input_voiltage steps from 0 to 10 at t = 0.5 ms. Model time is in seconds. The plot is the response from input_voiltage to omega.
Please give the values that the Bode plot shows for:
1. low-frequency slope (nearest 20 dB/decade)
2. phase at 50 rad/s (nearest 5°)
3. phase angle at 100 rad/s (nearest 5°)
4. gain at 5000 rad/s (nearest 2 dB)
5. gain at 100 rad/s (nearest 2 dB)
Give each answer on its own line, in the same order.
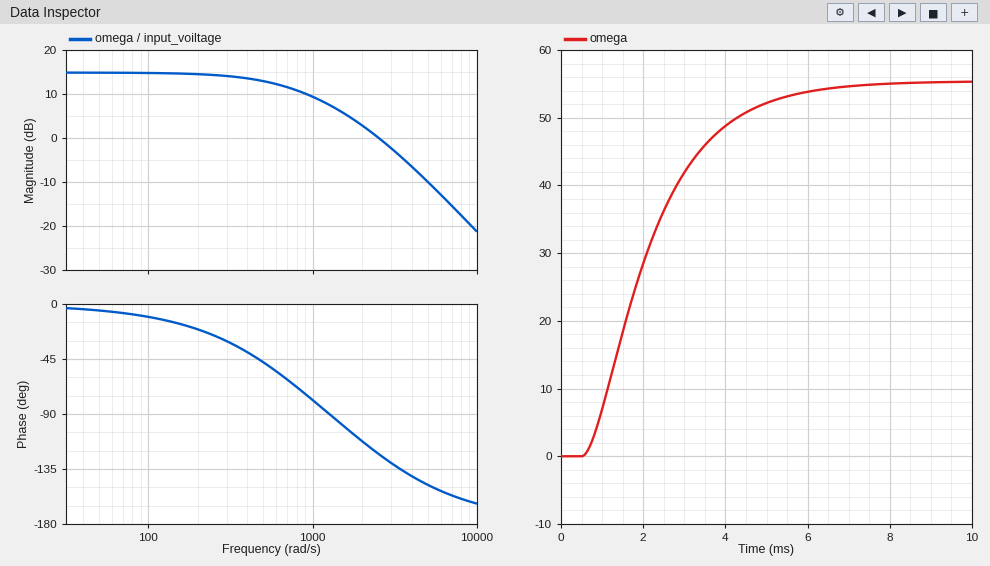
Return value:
0 dB/decade
-5°
-10°
-10 dB
14 dB
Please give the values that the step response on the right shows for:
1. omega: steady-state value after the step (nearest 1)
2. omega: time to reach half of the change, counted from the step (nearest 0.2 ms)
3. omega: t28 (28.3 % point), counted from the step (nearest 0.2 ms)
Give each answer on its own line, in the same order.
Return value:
55
1.4 ms
0.8 ms
